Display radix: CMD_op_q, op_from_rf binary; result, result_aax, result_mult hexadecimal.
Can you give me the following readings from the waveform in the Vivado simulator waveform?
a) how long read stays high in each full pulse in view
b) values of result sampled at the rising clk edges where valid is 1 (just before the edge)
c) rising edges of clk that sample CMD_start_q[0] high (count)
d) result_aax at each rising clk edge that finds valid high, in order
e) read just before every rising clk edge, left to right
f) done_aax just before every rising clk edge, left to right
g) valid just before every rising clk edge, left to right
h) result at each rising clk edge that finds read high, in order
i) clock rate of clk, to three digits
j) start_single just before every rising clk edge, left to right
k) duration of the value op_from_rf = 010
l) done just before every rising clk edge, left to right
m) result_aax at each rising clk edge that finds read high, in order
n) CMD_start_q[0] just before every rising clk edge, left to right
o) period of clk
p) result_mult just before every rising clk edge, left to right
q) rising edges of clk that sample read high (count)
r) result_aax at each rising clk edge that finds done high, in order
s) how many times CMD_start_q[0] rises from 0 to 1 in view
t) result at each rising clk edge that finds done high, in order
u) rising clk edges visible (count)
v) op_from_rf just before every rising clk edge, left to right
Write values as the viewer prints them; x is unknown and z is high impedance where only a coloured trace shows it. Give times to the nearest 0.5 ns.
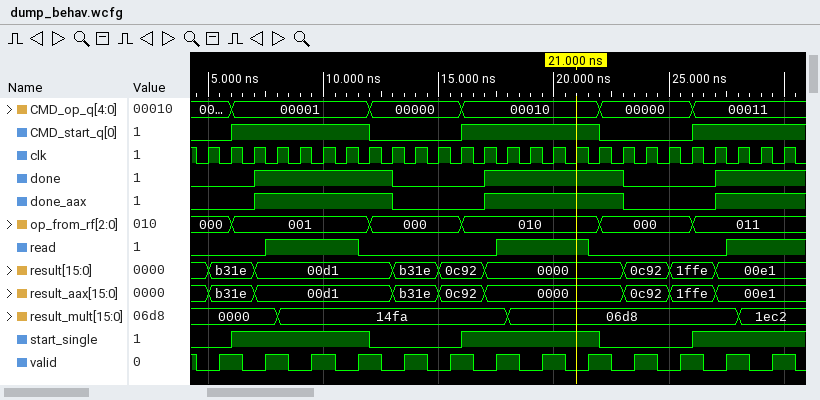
4 ns, 4 ns
b31e, 00d1, 00d1, 00d1, b31e, 0c92, 0000, 0000, 0000, 0c92, 1ffe, 00e1, 00e1
16
b31e, 00d1, 00d1, 00d1, b31e, 0c92, 0000, 0000, 0000, 0c92, 1ffe, 00e1, 00e1
0 0 0 1 1 1 1 0 0 0 0 0 0 1 1 1 1 0 0 0 0 0 0 1 1 1
0 0 0 1 1 1 1 1 1 0 0 0 0 1 1 1 1 1 1 0 0 0 0 1 1 1
0 1 0 1 0 1 0 1 0 1 0 1 0 1 0 1 0 1 0 1 0 1 0 1 0 1
00d1, 00d1, 00d1, 00d1, 0000, 0000, 0000, 0000, 00e1, 00e1, 00e1
1.00 GHz
0 0 1 1 1 1 1 1 0 0 0 0 1 1 1 1 1 1 0 0 0 0 1 1 1 1
6 ns
0 0 0 1 1 1 1 1 1 0 0 0 0 1 1 1 1 1 1 0 0 0 0 1 1 1
00d1, 00d1, 00d1, 00d1, 0000, 0000, 0000, 0000, 00e1, 00e1, 00e1
0 0 1 1 1 1 1 1 0 0 0 0 1 1 1 1 1 1 0 0 0 0 1 1 1 1
1 ns
0000, 0000, 0000, 0000, 14fa, 14fa, 14fa, 14fa, 14fa, 14fa, 14fa, 14fa, 14fa, 14fa, 06d8, 06d8, 06d8, 06d8, 06d8, 06d8, 06d8, 06d8, 06d8, 06d8, 1ec2, 1ec2
11
00d1, 00d1, 00d1, 00d1, 00d1, 00d1, 0000, 0000, 0000, 0000, 0000, 0000, 00e1, 00e1, 00e1
3
00d1, 00d1, 00d1, 00d1, 00d1, 00d1, 0000, 0000, 0000, 0000, 0000, 0000, 00e1, 00e1, 00e1
26
000, 000, 001, 001, 001, 001, 001, 001, 000, 000, 000, 000, 010, 010, 010, 010, 010, 010, 000, 000, 000, 000, 011, 011, 011, 011
